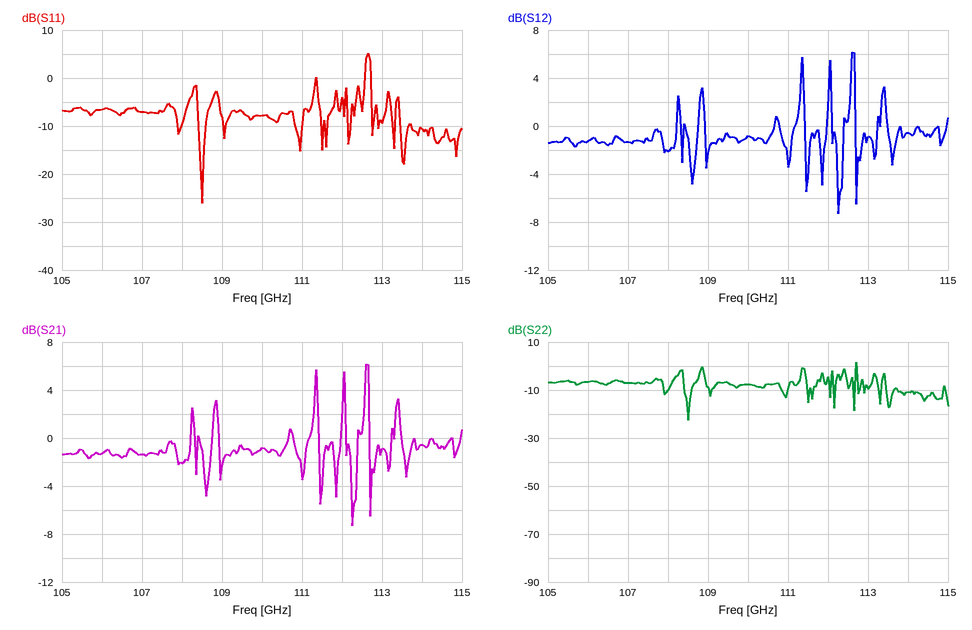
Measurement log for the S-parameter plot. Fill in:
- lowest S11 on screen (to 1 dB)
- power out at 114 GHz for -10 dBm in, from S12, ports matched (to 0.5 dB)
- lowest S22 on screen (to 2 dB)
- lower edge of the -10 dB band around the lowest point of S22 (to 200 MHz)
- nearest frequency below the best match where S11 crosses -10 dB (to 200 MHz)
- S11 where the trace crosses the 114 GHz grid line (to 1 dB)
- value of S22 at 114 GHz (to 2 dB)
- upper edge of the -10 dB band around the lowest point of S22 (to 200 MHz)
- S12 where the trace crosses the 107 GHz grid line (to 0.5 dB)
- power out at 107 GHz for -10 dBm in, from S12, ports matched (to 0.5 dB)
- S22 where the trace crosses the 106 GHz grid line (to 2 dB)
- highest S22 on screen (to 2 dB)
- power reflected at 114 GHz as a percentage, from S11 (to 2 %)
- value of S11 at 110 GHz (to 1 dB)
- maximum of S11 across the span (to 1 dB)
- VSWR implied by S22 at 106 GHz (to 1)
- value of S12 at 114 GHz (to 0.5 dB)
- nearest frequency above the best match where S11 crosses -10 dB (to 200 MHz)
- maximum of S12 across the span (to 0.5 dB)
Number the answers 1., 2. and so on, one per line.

1. -26 dB
2. -10.5 dBm
3. -22 dB
4. 108.4 GHz
5. 108.4 GHz
6. -11 dB
7. -10 dB
8. 108.6 GHz
9. -1.5 dB
10. -11.5 dBm
11. -6 dB
12. 2 dB
13. 8 %
14. -8 dB
15. 5 dB
16. 3
17. -0.5 dB
18. 108.6 GHz
19. 6.0 dB
